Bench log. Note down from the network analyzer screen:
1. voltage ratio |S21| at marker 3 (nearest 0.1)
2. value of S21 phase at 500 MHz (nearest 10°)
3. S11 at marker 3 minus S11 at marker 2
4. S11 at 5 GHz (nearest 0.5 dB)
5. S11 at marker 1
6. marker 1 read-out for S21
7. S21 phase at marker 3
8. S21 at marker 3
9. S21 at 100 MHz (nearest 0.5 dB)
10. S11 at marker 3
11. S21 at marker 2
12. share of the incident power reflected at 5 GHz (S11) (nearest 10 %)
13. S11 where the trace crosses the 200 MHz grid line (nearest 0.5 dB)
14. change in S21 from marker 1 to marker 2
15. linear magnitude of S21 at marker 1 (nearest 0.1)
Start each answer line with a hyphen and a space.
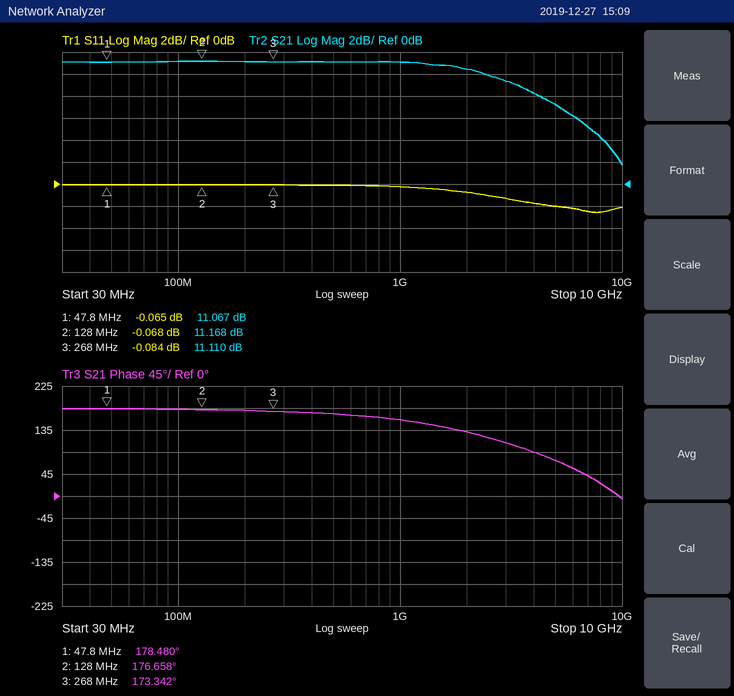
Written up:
- 3.6
- 170°
- -0.016 dB
- -2.0 dB
- -0.065 dB
- 11.067 dB
- 173.342°
- 11.110 dB
- 11.0 dB
- -0.084 dB
- 11.168 dB
- 60 %
- 0.0 dB
- 0.101 dB
- 3.6
